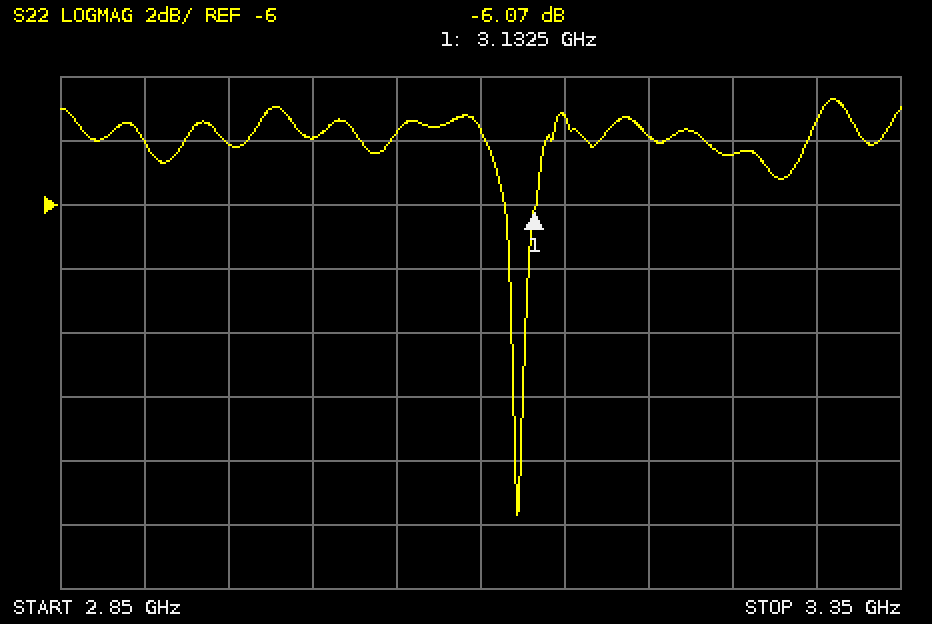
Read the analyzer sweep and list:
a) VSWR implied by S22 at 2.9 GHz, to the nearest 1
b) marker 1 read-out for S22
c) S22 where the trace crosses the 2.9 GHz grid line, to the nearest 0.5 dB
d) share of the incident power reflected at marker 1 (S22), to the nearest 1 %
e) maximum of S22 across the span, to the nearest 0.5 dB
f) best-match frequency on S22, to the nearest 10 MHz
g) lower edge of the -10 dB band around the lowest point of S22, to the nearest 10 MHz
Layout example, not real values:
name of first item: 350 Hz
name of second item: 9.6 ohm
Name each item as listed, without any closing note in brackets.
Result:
VSWR implied by S22 at 2.9 GHz, to the nearest 1: 4
marker 1 read-out for S22: -6.07 dB
S22 where the trace crosses the 2.9 GHz grid line, to the nearest 0.5 dB: -4.0 dB
share of the incident power reflected at marker 1 (S22), to the nearest 1 %: 25 %
maximum of S22 across the span, to the nearest 0.5 dB: -2.5 dB
best-match frequency on S22, to the nearest 10 MHz: 3.12 GHz
lower edge of the -10 dB band around the lowest point of S22, to the nearest 10 MHz: 3.12 GHz
